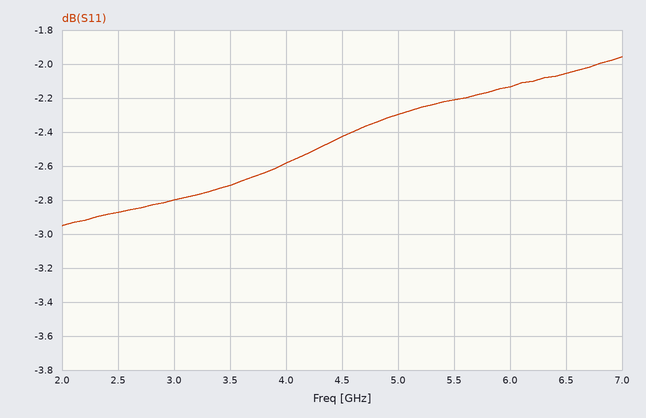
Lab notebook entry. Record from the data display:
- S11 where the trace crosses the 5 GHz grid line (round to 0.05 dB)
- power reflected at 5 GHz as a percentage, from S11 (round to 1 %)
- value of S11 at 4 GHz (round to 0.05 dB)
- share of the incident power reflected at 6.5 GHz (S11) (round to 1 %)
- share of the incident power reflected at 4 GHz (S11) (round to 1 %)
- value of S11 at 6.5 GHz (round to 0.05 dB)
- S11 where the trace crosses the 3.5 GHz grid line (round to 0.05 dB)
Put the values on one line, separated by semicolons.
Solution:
-2.30 dB; 59 %; -2.60 dB; 62 %; 55 %; -2.05 dB; -2.70 dB
